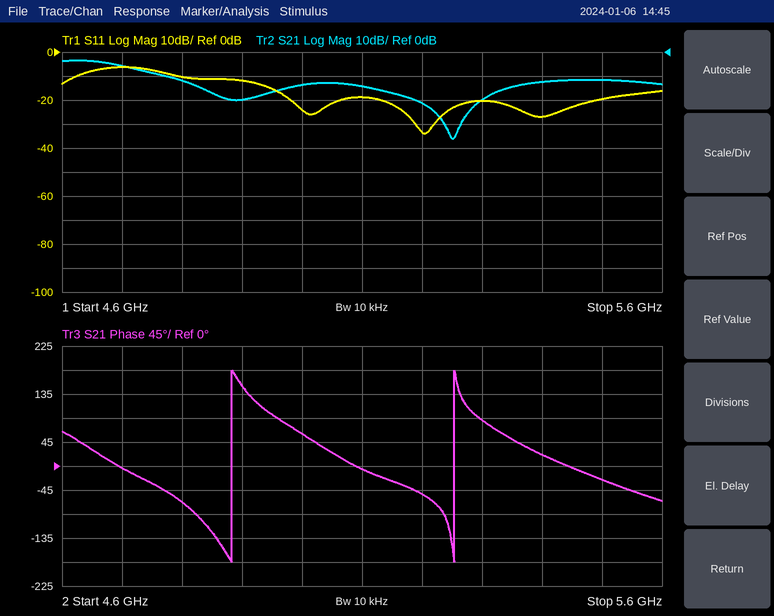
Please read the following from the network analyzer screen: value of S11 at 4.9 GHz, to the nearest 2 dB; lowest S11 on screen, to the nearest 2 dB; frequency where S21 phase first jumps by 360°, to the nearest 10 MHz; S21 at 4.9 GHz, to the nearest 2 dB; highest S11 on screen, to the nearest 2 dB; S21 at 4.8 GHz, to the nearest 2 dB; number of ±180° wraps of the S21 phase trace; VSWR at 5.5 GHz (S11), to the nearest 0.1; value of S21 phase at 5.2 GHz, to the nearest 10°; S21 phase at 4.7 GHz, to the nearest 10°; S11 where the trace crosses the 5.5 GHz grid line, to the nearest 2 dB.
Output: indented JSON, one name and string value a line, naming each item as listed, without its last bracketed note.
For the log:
{
  "value of S11 at 4.9 GHz, to the nearest 2 dB": "-12 dB",
  "lowest S11 on screen, to the nearest 2 dB": "-34 dB",
  "frequency where S21 phase first jumps by 360°, to the nearest 10 MHz": "4.88 GHz",
  "S21 at 4.9 GHz, to the nearest 2 dB": "-20 dB",
  "highest S11 on screen, to the nearest 2 dB": "-6 dB",
  "S21 at 4.8 GHz, to the nearest 2 dB": "-12 dB",
  "number of ±180° wraps of the S21 phase trace": "2",
  "VSWR at 5.5 GHz (S11), to the nearest 0.1": "1.2",
  "value of S21 phase at 5.2 GHz, to the nearest 10°": "-50°",
  "S21 phase at 4.7 GHz, to the nearest 10°": "0°",
  "S11 where the trace crosses the 5.5 GHz grid line, to the nearest 2 dB": "-20 dB"
}
